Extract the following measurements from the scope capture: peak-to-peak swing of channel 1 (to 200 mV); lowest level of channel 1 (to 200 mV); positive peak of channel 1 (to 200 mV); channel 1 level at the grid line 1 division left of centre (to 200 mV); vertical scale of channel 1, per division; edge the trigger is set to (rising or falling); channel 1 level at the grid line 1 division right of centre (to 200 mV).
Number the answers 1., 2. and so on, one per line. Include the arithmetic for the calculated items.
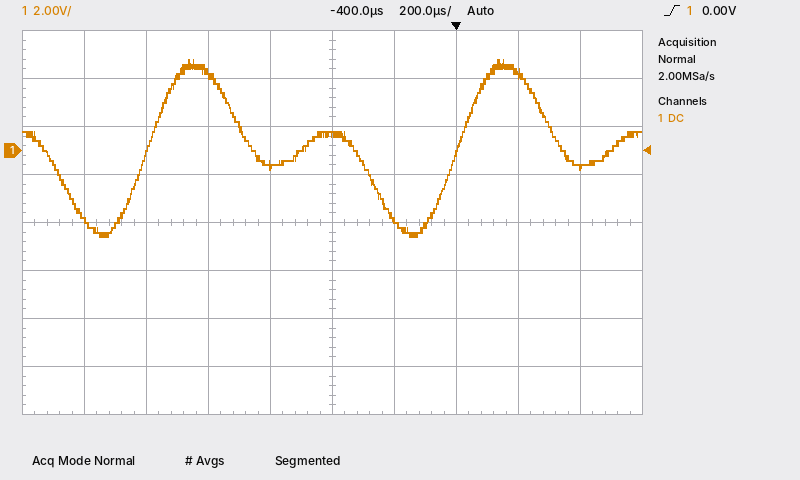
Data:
1. 3.8 V − (-3.6 V) = 7.4 V
2. -3.6 V
3. 3.8 V
4. -600 mV
5. 2 V
6. rising
7. -2.8 V
